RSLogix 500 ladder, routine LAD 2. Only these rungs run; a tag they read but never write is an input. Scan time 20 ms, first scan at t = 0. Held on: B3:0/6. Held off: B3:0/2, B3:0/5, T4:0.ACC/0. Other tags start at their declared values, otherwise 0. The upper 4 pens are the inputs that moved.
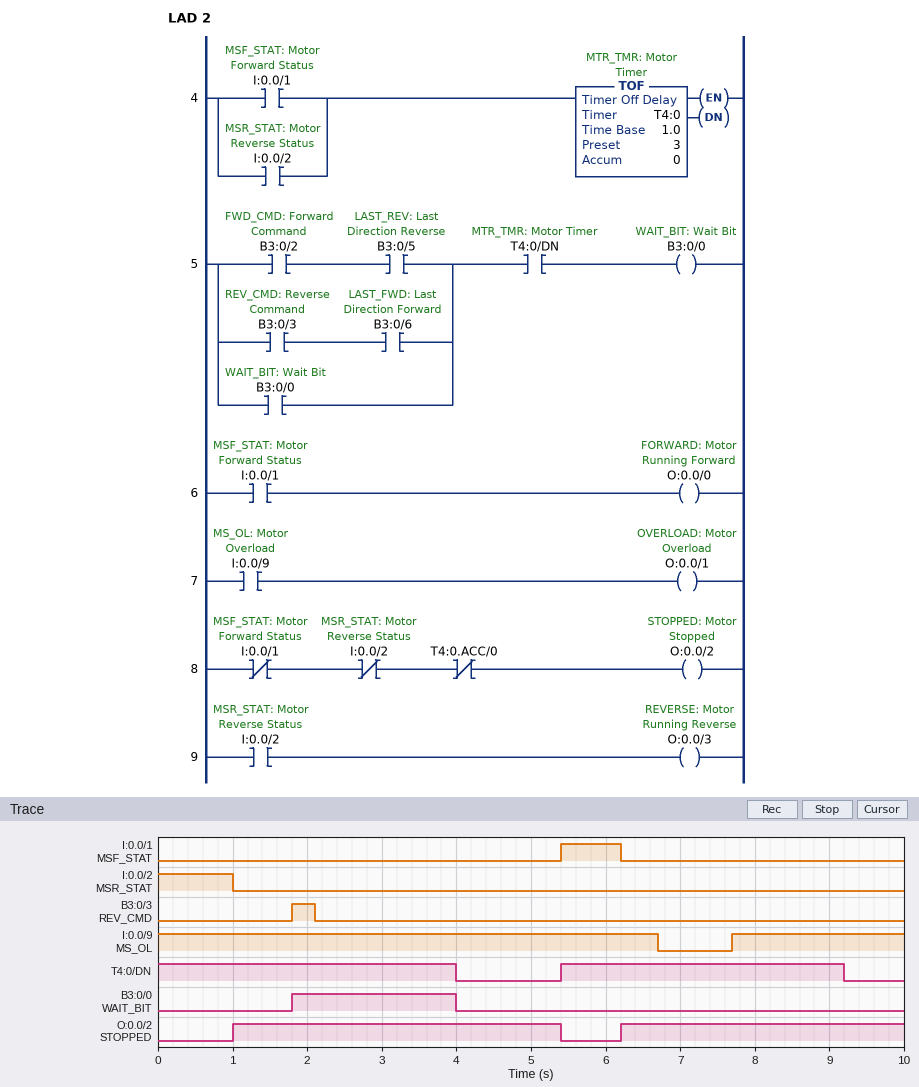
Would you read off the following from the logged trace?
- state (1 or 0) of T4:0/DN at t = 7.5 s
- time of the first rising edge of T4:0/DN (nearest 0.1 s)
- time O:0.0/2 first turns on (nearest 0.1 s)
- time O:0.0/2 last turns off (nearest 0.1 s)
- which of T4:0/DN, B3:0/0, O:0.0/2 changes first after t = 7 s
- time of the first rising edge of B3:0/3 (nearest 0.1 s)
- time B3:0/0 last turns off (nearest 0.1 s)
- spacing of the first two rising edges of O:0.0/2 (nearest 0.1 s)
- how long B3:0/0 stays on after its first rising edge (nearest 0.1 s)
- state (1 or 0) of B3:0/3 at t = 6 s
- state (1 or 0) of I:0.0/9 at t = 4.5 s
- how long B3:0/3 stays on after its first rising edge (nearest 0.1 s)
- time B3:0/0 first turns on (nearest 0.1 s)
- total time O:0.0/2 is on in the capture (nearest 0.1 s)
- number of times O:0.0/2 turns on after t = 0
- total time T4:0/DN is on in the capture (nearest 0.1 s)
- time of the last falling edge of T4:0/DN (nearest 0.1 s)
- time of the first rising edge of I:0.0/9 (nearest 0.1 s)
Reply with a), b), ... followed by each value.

a) 1
b) 5.4 s
c) 1.0 s
d) 5.4 s
e) T4:0/DN
f) 1.8 s
g) 4.0 s
h) 5.2 s
i) 2.2 s
j) 0
k) 1
l) 0.3 s
m) 1.8 s
n) 8.2 s
o) 2
p) 7.8 s
q) 9.2 s
r) 7.7 s
